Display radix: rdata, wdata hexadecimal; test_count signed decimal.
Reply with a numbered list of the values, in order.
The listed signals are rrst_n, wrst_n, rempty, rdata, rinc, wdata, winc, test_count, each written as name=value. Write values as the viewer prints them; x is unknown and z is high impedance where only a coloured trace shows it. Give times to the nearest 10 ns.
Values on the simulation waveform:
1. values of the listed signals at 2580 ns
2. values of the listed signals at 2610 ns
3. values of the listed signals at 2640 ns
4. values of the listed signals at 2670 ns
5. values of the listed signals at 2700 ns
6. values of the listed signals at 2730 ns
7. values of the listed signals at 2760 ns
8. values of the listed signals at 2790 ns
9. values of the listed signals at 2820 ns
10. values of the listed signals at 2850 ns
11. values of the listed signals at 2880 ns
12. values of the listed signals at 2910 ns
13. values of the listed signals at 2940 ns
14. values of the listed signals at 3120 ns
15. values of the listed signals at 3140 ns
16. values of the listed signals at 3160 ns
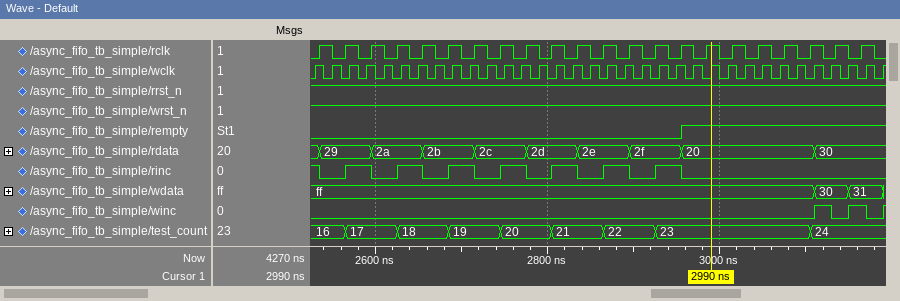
1. rrst_n=1, wrst_n=1, rempty=0, rdata=29, rinc=1, wdata=ff, winc=0, test_count=17
2. rrst_n=1, wrst_n=1, rempty=0, rdata=2a, rinc=0, wdata=ff, winc=0, test_count=17
3. rrst_n=1, wrst_n=1, rempty=0, rdata=2a, rinc=1, wdata=ff, winc=0, test_count=18
4. rrst_n=1, wrst_n=1, rempty=0, rdata=2b, rinc=0, wdata=ff, winc=0, test_count=18
5. rrst_n=1, wrst_n=1, rempty=0, rdata=2b, rinc=1, wdata=ff, winc=0, test_count=19
6. rrst_n=1, wrst_n=1, rempty=0, rdata=2c, rinc=0, wdata=ff, winc=0, test_count=19
7. rrst_n=1, wrst_n=1, rempty=0, rdata=2c, rinc=1, wdata=ff, winc=0, test_count=20
8. rrst_n=1, wrst_n=1, rempty=0, rdata=2d, rinc=0, wdata=ff, winc=0, test_count=20
9. rrst_n=1, wrst_n=1, rempty=0, rdata=2d, rinc=1, wdata=ff, winc=0, test_count=21
10. rrst_n=1, wrst_n=1, rempty=0, rdata=2e, rinc=0, wdata=ff, winc=0, test_count=21
11. rrst_n=1, wrst_n=1, rempty=0, rdata=2e, rinc=1, wdata=ff, winc=0, test_count=22
12. rrst_n=1, wrst_n=1, rempty=0, rdata=2f, rinc=0, wdata=ff, winc=0, test_count=22
13. rrst_n=1, wrst_n=1, rempty=0, rdata=2f, rinc=1, wdata=ff, winc=0, test_count=23
14. rrst_n=1, wrst_n=1, rempty=1, rdata=30, rinc=0, wdata=30, winc=1, test_count=24
15. rrst_n=1, wrst_n=1, rempty=1, rdata=30, rinc=0, wdata=30, winc=0, test_count=24
16. rrst_n=1, wrst_n=1, rempty=1, rdata=30, rinc=0, wdata=31, winc=1, test_count=24
